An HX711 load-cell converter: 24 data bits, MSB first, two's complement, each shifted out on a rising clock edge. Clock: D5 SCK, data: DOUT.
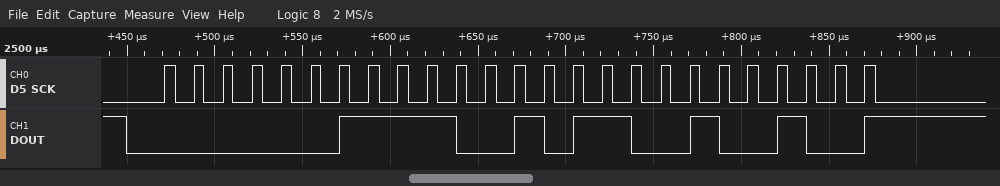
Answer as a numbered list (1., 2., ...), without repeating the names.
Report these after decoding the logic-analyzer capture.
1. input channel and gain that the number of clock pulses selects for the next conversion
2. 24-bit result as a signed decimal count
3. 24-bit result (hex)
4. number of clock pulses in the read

1. channel A, gain 128
2. 248612
3. 0x03CB24
4. 25
